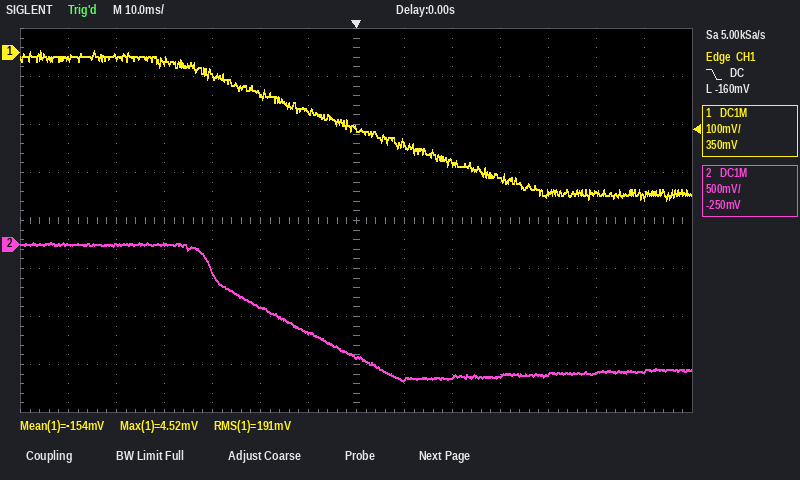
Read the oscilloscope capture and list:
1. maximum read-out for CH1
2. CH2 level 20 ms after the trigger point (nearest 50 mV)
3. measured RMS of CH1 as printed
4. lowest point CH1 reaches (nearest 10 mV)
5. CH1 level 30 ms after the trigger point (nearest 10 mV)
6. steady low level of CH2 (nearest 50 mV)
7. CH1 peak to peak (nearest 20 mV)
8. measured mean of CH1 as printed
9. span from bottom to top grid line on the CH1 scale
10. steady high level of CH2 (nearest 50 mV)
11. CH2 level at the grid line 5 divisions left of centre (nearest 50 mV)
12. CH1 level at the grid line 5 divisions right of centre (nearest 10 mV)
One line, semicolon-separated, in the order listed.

4.52 mV; -1.40 V; 191 mV; -310 mV; -260 mV; -1.35 V; 320 mV; -154 mV; 800 mV; 0 mV; 0 mV; -290 mV
